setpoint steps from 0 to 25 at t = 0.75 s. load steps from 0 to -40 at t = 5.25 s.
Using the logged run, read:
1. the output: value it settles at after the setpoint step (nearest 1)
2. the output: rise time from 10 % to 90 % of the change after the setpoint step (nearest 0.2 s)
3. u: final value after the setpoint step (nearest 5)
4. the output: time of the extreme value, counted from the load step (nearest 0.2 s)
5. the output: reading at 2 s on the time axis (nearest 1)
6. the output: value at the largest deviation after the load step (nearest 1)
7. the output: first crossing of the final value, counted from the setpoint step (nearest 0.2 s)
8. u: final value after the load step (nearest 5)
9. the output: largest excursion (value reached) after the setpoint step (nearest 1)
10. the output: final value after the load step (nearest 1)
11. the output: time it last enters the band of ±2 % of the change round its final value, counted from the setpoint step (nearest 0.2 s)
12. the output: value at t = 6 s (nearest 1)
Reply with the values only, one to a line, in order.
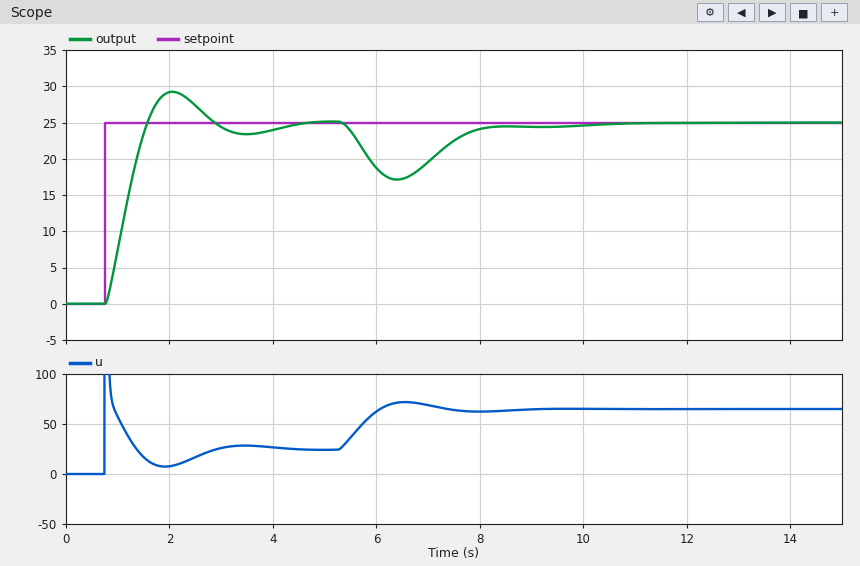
25
0.6 s
25
1.2 s
29
17
0.8 s
65
29
25
3.6 s
19
